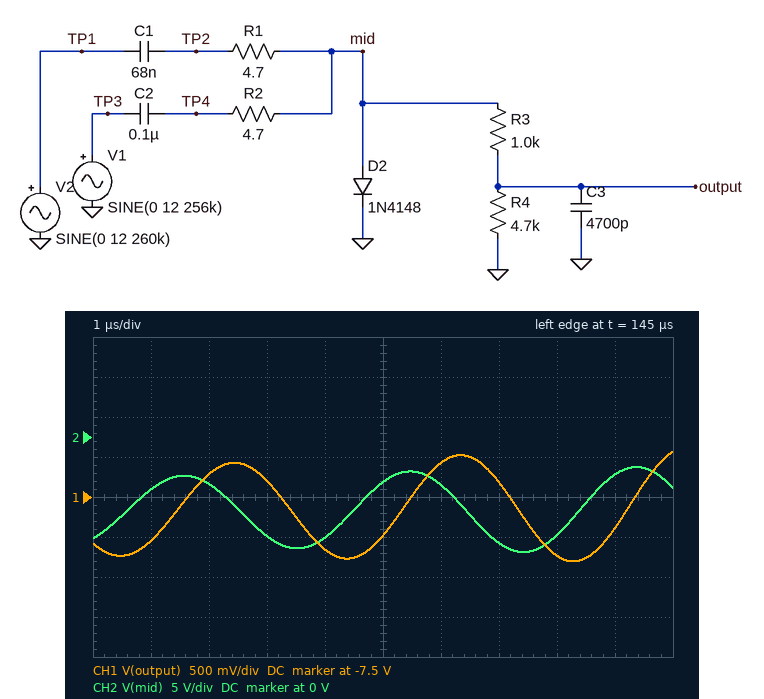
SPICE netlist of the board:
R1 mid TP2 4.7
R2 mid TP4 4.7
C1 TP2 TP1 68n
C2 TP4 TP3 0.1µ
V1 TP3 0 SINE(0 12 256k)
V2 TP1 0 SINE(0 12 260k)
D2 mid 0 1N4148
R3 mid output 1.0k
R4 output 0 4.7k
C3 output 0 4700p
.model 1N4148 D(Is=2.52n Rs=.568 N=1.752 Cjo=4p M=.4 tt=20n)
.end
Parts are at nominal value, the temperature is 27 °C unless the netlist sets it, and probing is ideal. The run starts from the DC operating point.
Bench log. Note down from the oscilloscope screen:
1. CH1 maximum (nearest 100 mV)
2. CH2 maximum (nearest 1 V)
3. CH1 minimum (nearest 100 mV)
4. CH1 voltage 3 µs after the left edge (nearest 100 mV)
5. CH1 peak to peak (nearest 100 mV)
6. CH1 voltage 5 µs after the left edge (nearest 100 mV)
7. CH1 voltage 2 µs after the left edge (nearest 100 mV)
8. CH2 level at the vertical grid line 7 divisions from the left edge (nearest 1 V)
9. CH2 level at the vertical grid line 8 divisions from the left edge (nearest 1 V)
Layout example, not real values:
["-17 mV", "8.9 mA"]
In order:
["-6.9 V", "-4 V", "-8.3 V", "-7.3 V", "1.4 V", "-8.0 V", "-7.2 V", "-13 V", "-12 V"]
